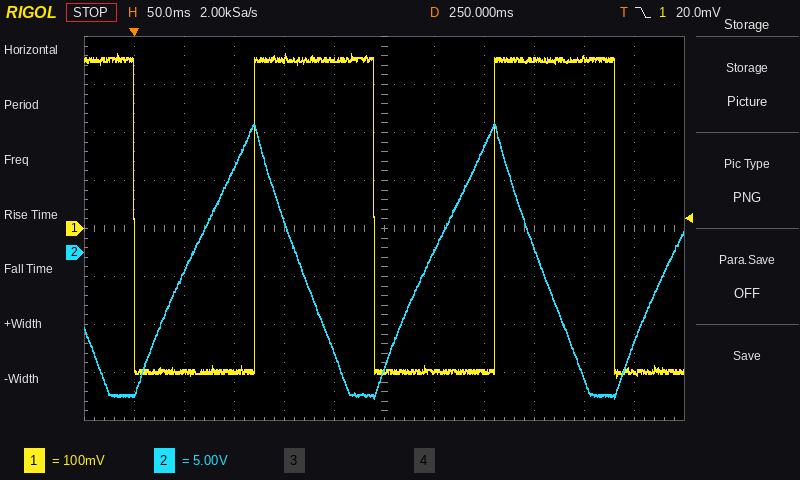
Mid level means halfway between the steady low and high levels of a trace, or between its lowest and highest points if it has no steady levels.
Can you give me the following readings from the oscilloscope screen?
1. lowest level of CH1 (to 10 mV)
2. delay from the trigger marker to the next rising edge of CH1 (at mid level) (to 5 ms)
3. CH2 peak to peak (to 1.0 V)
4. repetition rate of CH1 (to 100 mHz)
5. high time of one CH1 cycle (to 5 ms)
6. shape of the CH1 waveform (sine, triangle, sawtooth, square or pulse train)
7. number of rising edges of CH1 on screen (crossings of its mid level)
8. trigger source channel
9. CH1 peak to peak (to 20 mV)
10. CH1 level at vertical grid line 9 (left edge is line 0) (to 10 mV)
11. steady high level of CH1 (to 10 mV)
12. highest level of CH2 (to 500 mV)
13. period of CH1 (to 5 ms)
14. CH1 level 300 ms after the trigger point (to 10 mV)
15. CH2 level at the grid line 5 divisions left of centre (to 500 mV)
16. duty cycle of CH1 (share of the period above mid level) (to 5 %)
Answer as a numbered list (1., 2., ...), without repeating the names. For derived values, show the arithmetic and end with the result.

1. -310 mV
2. 120 ms
3. 29.0 V
4. 1 / 240 ms ≈ 4.2 Hz
5. 120 ms
6. square
7. 2
8. CH1
9. 680 mV
10. 350 mV
11. 350 mV
12. 13.5 V
13. 240 ms
14. -300 mV
15. -14.5 V
16. 120 ms / 240 ms ≈ 50 %
